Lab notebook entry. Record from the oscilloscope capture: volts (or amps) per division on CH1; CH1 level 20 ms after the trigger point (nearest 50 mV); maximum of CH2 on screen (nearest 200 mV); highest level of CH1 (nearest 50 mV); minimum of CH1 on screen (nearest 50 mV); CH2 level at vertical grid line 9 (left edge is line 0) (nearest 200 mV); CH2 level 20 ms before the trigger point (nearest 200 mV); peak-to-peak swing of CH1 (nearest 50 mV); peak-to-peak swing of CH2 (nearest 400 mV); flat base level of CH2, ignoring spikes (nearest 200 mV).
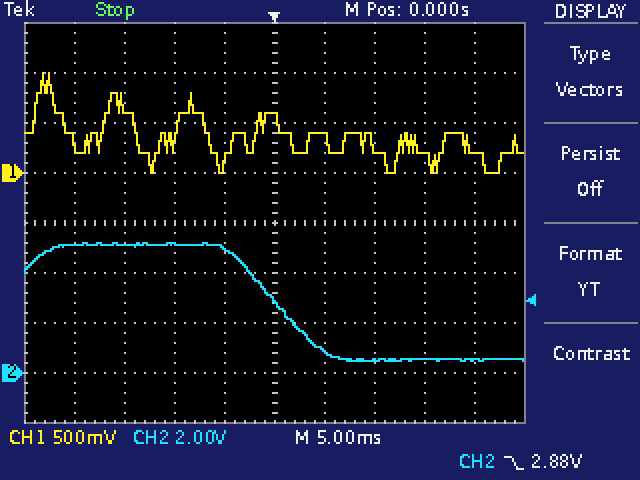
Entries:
500 mV
200 mV
5.2 V
1.00 V
0 mV
600 mV
5.2 V
1.00 V
4.8 V
600 mV
